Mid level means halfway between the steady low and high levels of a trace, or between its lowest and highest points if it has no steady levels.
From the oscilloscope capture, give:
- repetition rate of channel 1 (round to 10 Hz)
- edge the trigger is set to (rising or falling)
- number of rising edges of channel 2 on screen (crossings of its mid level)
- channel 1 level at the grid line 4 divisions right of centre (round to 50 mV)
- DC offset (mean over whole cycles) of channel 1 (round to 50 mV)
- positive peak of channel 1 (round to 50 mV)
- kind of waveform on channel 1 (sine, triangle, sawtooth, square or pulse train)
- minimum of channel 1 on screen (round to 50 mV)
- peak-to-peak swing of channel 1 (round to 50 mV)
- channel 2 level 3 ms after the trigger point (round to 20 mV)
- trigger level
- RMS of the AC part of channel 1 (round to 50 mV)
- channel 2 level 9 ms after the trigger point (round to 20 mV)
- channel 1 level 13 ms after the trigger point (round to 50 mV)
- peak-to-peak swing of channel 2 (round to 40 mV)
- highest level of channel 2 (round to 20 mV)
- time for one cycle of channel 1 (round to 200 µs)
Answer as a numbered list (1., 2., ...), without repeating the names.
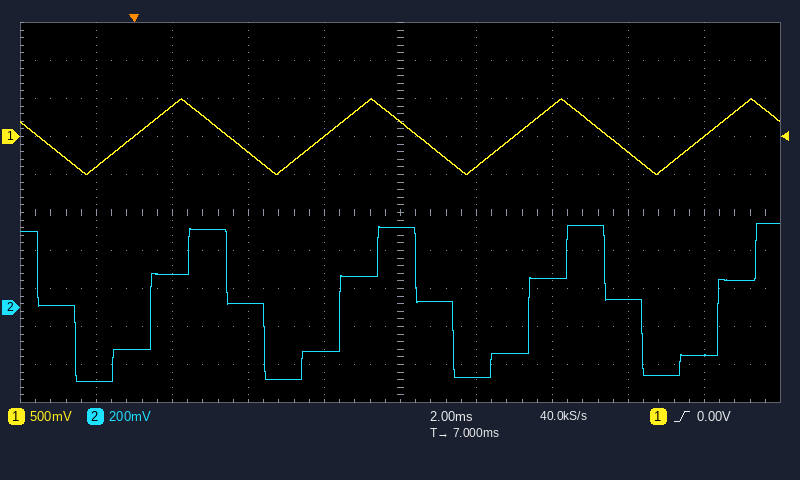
1. 200 Hz
2. rising
3. 4
4. 0 mV
5. 0 mV
6. 500 mV
7. triangle
8. -500 mV
9. 1.00 V
10. 20 mV
11. 0.00 V
12. 300 mV
13. -360 mV
14. -200 mV
15. 840 mV
16. 440 mV
17. 5.0 ms
